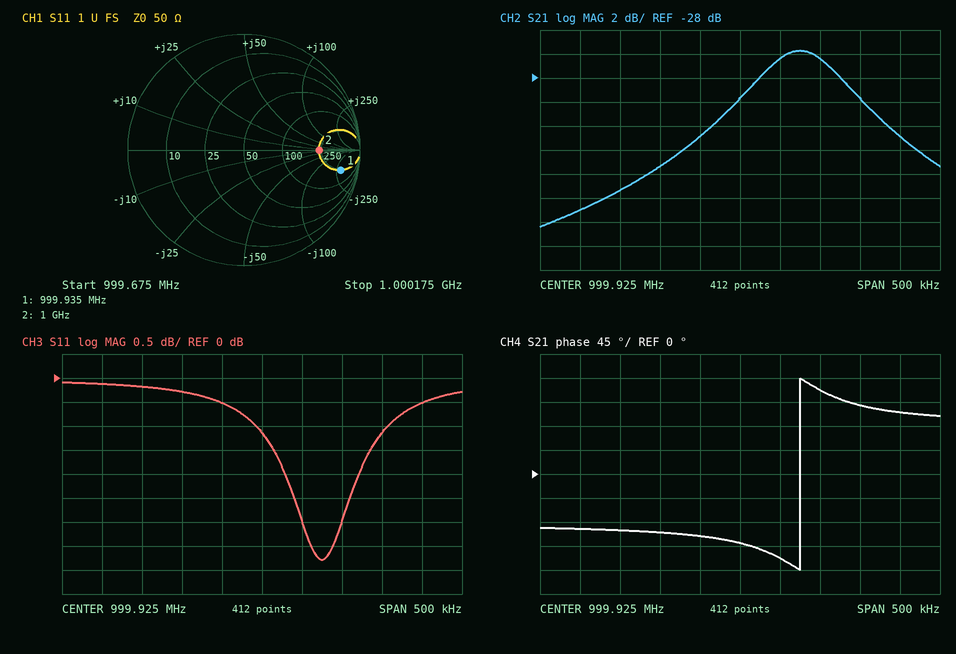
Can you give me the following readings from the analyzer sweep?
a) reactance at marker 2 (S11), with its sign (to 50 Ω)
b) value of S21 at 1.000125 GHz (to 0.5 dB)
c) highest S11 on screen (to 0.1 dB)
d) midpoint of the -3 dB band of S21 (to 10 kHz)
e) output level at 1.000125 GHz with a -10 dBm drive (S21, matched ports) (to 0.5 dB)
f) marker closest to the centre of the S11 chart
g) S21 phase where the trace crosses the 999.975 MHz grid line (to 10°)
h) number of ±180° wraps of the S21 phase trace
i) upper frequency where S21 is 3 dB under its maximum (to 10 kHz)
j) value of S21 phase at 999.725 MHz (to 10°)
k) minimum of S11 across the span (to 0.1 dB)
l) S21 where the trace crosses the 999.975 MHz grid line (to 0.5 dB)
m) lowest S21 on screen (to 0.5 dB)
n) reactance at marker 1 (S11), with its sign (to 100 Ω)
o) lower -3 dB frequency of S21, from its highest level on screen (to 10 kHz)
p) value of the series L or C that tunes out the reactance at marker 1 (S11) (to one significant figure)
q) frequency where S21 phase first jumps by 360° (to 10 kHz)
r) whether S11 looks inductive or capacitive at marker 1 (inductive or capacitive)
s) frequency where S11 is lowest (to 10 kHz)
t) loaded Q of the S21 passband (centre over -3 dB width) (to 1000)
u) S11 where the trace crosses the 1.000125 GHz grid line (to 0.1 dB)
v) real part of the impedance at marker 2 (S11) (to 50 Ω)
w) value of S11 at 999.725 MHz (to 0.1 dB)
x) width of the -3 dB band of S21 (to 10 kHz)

0 Ω
-33.0 dB
-0.1 dB
1.00000 GHz
-43.0 dBm
marker 2
-160°
1
1.00006 GHz
-100°
-3.8 dB
-26.5 dB
-40.5 dB
-300 Ω
999.94 MHz
50 nH
1.00000 GHz
capacitive
1.00000 GHz
8000
-0.5 dB
250 Ω
-0.1 dB
120 kHz
